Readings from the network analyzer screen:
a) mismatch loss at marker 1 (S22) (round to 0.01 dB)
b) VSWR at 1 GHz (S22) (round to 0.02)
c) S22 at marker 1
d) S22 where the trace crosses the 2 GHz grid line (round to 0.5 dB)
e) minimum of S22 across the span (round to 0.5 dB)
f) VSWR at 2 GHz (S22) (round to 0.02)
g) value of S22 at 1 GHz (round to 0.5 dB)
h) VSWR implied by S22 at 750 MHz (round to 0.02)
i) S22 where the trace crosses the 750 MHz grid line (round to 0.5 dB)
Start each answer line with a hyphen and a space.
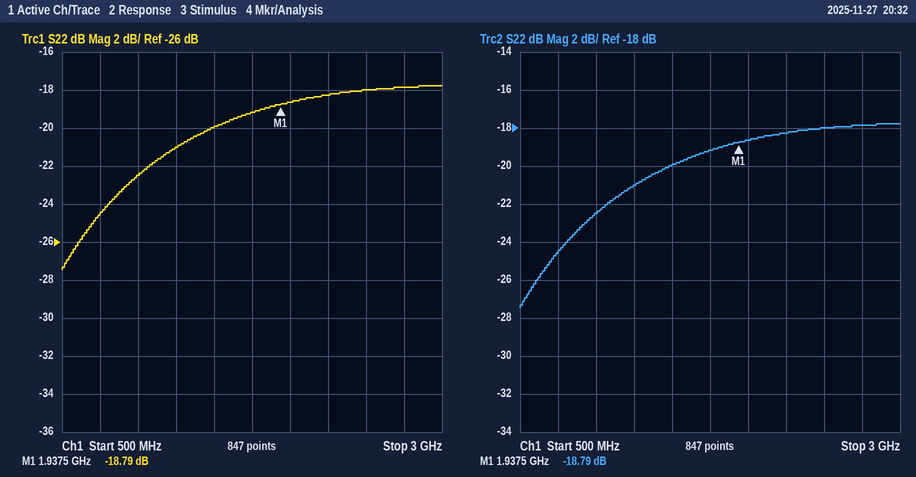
- 0.06 dB
- 1.16
- -18.79 dB
- -18.5 dB
- -27.5 dB
- 1.26
- -22.5 dB
- 1.12
- -24.5 dB
